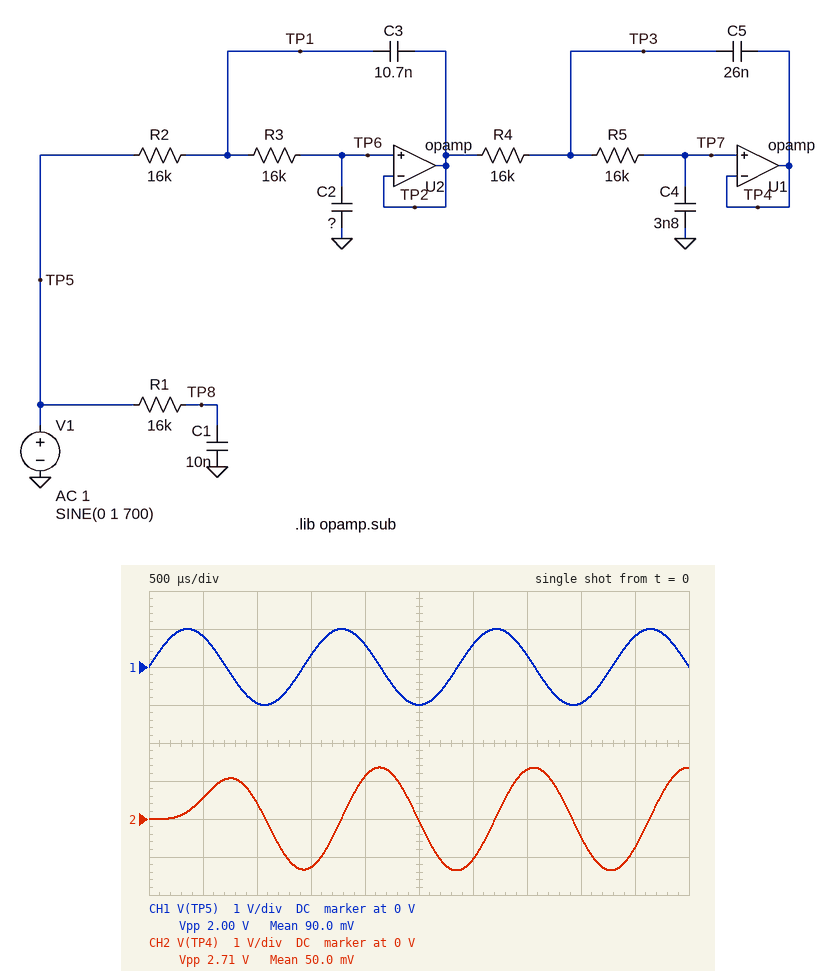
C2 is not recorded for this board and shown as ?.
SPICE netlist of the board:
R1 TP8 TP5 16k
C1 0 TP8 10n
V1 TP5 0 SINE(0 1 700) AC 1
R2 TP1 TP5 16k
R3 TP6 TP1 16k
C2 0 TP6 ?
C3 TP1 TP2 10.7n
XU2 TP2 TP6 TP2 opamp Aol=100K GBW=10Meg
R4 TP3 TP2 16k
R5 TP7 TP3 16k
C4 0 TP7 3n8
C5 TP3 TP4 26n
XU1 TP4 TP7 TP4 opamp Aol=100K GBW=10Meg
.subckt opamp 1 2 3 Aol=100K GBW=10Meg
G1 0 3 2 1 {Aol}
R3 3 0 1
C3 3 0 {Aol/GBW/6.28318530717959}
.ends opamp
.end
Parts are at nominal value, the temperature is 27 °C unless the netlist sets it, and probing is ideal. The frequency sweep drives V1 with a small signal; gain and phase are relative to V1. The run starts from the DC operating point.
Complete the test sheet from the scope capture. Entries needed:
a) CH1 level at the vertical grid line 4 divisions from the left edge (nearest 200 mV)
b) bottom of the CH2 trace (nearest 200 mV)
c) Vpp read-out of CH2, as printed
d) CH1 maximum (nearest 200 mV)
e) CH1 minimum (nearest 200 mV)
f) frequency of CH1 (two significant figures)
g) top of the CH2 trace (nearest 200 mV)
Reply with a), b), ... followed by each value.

a) 600 mV
b) -1.4 V
c) 2.71 V
d) 1.0 V
e) -1.0 V
f) 700 Hz
g) 1.4 V
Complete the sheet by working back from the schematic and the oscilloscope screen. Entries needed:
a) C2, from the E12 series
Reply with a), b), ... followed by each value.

a) 4.7 nF
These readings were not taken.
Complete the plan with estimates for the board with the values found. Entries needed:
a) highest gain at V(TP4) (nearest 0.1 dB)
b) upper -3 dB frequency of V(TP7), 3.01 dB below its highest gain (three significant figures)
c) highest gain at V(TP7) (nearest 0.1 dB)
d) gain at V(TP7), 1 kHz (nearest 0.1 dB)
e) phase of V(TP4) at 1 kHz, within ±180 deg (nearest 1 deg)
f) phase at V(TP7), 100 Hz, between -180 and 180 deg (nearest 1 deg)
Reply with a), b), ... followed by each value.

a) 2.9 dB
b) 1.13 kHz
c) 2.9 dB
d) 1.8 dB
e) -152 deg
f) -10 deg
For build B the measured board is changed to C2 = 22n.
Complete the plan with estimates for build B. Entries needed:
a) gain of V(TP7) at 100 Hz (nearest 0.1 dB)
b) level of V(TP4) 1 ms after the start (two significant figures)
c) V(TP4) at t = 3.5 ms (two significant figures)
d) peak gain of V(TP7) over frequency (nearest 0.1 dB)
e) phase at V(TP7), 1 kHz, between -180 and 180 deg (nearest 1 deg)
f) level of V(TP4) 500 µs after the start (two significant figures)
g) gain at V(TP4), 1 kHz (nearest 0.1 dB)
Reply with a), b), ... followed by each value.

a) -0.5 dB
b) 470 mV
c) 170 mV
d) 0 dB
e) 163 deg
f) 160 mV
g) -11.0 dB
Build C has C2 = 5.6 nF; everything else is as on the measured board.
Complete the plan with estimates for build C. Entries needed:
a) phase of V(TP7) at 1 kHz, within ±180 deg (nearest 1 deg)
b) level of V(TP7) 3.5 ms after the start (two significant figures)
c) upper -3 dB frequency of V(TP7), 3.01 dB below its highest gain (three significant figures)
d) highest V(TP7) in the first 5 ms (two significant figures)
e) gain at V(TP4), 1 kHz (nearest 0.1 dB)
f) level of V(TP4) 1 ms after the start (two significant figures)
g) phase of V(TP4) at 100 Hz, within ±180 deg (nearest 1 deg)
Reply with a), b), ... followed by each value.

a) -161 deg
b) 1.2 V
c) 1.10 kHz
d) 1.3 V
e) 0.8 dB
f) 500 mV
g) -11 deg
